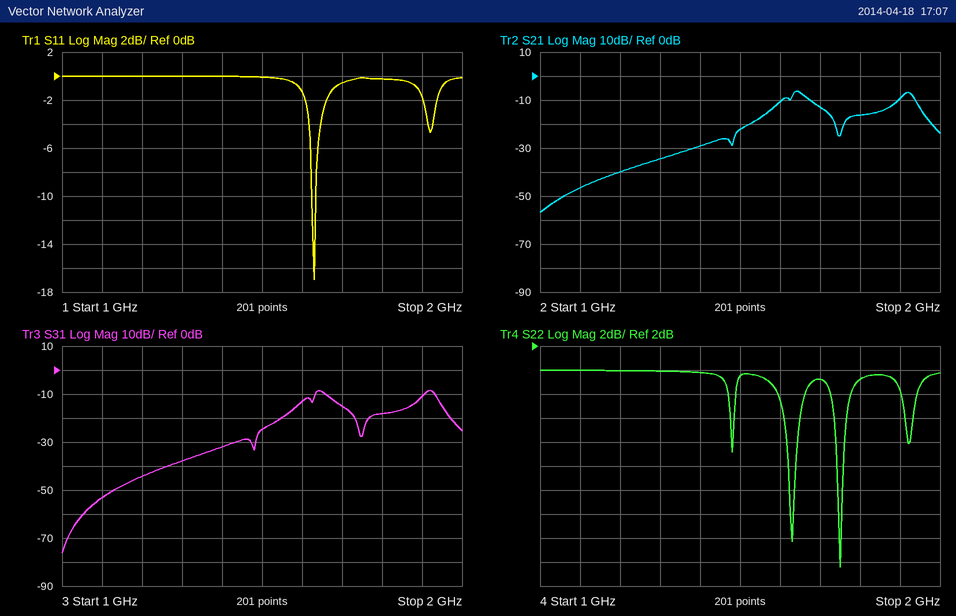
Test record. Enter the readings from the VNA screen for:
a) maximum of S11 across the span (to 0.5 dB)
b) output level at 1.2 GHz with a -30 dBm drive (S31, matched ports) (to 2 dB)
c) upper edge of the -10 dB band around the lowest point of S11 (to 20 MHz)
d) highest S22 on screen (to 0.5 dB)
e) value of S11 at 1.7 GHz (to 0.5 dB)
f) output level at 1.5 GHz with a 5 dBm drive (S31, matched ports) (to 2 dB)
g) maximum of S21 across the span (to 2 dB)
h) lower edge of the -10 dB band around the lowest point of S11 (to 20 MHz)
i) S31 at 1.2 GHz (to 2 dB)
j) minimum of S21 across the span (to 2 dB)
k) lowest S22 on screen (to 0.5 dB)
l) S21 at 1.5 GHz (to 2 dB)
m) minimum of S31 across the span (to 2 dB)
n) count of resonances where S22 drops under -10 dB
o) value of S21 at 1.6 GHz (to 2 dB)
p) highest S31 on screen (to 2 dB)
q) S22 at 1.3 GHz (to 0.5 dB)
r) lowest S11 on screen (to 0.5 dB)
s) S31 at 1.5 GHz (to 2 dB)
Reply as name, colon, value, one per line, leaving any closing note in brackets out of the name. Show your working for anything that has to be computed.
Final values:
maximum of S11 across the span: 0.0 dB
output level at 1.2 GHz with a -30 dBm drive (S31, matched ports): -30 dBm + (-44 dB) = -74 dBm
upper edge of the -10 dB band around the lowest point of S11: 1.64 GHz
highest S22 on screen: 0.0 dB
value of S11 at 1.7 GHz: -0.5 dB
output level at 1.5 GHz with a 5 dBm drive (S31, matched ports): 5 dBm + (-24 dB) = -20 dBm
maximum of S21 across the span: -6 dB
lower edge of the -10 dB band around the lowest point of S11: 1.62 GHz
S31 at 1.2 GHz: -44 dB
minimum of S21 across the span: -56 dB
lowest S22 on screen: -16.5 dB
S21 at 1.5 GHz: -22 dB
minimum of S31 across the span: -76 dB
count of resonances where S22 drops under -10 dB: 2
value of S21 at 1.6 GHz: -10 dB
highest S31 on screen: -8 dB
S22 at 1.3 GHz: 0.0 dB
lowest S11 on screen: -17.0 dB
S31 at 1.5 GHz: -24 dB
